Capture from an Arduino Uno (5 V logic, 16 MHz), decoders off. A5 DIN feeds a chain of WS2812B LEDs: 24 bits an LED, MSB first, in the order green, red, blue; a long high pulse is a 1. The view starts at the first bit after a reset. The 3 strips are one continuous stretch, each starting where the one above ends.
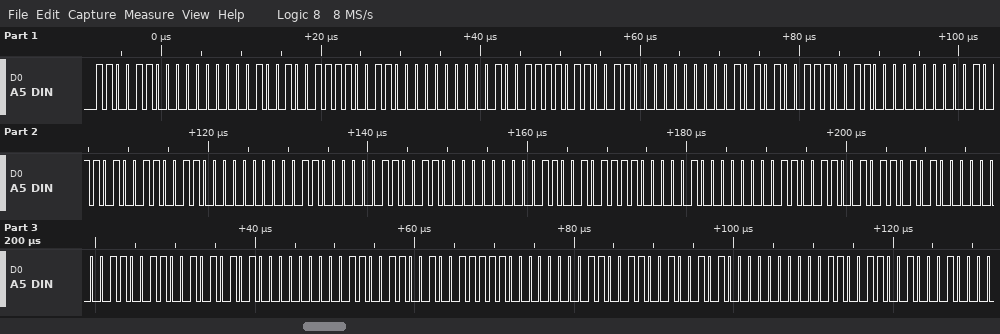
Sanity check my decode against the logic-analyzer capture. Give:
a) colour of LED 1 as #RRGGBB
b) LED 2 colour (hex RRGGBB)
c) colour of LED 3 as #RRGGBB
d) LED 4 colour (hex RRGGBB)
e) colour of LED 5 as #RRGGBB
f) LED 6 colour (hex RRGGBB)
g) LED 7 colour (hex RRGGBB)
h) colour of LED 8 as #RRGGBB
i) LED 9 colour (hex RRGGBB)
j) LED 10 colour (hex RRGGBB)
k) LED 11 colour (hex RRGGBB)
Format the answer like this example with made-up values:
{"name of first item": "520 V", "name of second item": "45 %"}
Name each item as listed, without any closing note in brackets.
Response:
{"colour of LED 1 as #RRGGBB": "#00CC93", "LED 2 colour": "#00CC9E", "colour of LED 3 as #RRGGBB": "#00CCA9", "LED 4 colour": "#00CCB4", "colour of LED 5 as #RRGGBB": "#00CCC0", "LED 6 colour": "#00CCCB", "LED 7 colour": "#00C1CC", "colour of LED 8 as #RRGGBB": "#00B5CC", "LED 9 colour": "#00AACC", "LED 10 colour": "#009FCC", "LED 11 colour": "#0094CC"}
